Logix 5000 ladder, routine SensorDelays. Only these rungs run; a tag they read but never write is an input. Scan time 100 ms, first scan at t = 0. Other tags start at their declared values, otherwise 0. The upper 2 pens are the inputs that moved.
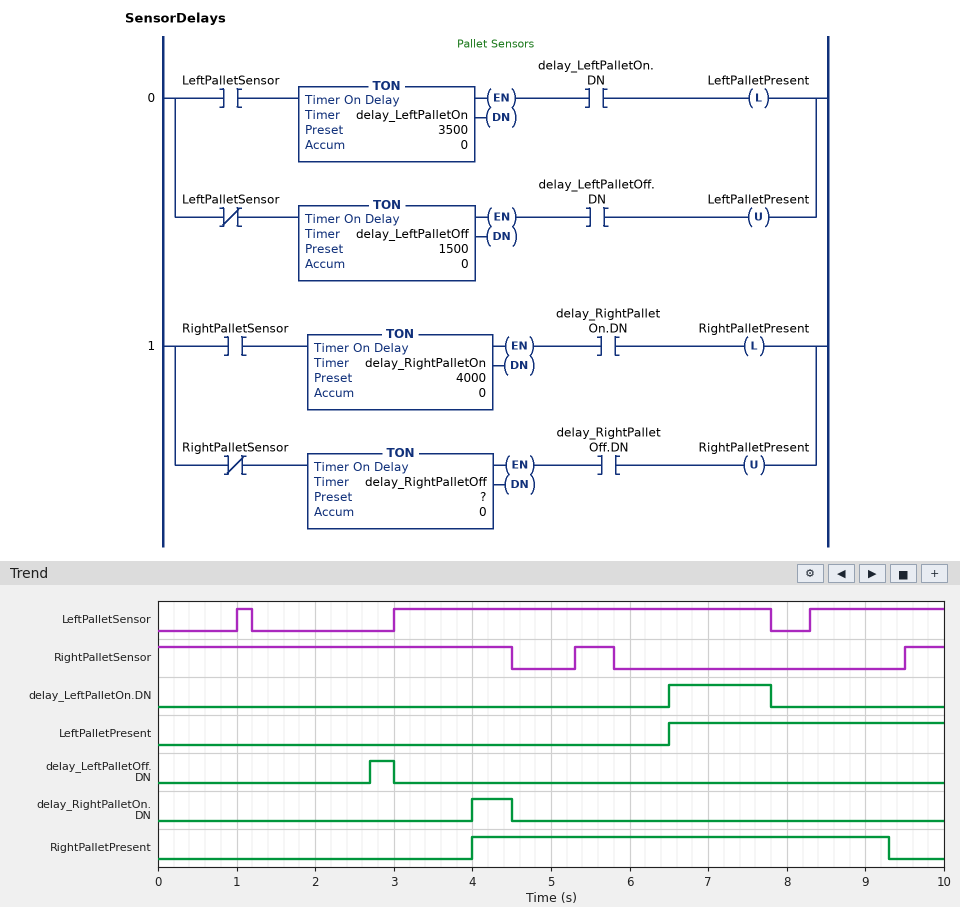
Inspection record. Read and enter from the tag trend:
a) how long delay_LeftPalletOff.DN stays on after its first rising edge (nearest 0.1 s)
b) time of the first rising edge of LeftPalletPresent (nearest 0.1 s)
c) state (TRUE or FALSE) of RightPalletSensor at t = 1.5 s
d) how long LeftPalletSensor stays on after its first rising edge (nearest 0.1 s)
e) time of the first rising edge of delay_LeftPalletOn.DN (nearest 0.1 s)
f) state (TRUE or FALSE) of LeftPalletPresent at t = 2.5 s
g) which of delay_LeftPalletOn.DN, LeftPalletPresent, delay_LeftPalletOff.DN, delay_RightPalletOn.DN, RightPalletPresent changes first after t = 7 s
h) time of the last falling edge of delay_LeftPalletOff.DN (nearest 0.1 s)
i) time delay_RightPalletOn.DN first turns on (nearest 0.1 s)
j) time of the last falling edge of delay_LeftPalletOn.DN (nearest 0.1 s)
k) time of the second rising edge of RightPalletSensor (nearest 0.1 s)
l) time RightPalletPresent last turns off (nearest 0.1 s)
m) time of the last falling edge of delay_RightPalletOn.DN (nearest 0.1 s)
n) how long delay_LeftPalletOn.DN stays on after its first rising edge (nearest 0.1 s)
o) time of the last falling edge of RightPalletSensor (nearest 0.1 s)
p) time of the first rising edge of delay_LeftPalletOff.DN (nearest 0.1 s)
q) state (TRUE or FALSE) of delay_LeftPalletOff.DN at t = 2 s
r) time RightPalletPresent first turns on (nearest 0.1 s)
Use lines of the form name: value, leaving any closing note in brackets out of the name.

how long delay_LeftPalletOff.DN stays on after its first rising edge: 0.3 s
time of the first rising edge of LeftPalletPresent: 6.5 s
state (TRUE or FALSE) of RightPalletSensor at t = 1.5 s: TRUE
how long LeftPalletSensor stays on after its first rising edge: 0.2 s
time of the first rising edge of delay_LeftPalletOn.DN: 6.5 s
state (TRUE or FALSE) of LeftPalletPresent at t = 2.5 s: FALSE
which of delay_LeftPalletOn.DN, LeftPalletPresent, delay_LeftPalletOff.DN, delay_RightPalletOn.DN, RightPalletPresent changes first after t = 7 s: delay_LeftPalletOn.DN
time of the last falling edge of delay_LeftPalletOff.DN: 3.0 s
time delay_RightPalletOn.DN first turns on: 4.0 s
time of the last falling edge of delay_LeftPalletOn.DN: 7.8 s
time of the second rising edge of RightPalletSensor: 9.5 s
time RightPalletPresent last turns off: 9.3 s
time of the last falling edge of delay_RightPalletOn.DN: 4.5 s
how long delay_LeftPalletOn.DN stays on after its first rising edge: 1.3 s
time of the last falling edge of RightPalletSensor: 5.8 s
time of the first rising edge of delay_LeftPalletOff.DN: 2.7 s
state (TRUE or FALSE) of delay_LeftPalletOff.DN at t = 2 s: FALSE
time RightPalletPresent first turns on: 4.0 s
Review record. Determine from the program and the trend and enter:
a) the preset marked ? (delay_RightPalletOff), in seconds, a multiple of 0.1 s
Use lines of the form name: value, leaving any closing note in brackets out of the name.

the preset marked ? (delay_RightPalletOff), in seconds, a multiple of 0.1 s: 3.5 s
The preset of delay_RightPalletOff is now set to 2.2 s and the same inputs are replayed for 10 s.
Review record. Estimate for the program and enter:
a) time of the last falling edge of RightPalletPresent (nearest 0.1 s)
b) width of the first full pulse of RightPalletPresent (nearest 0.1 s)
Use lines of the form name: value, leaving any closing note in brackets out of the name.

time of the last falling edge of RightPalletPresent: 8.0 s
width of the first full pulse of RightPalletPresent: 4.0 s
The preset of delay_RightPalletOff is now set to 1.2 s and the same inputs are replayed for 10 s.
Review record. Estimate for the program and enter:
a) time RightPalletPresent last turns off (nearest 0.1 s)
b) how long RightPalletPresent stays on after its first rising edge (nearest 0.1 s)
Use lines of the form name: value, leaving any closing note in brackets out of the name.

time RightPalletPresent last turns off: 7.0 s
how long RightPalletPresent stays on after its first rising edge: 3.0 s
